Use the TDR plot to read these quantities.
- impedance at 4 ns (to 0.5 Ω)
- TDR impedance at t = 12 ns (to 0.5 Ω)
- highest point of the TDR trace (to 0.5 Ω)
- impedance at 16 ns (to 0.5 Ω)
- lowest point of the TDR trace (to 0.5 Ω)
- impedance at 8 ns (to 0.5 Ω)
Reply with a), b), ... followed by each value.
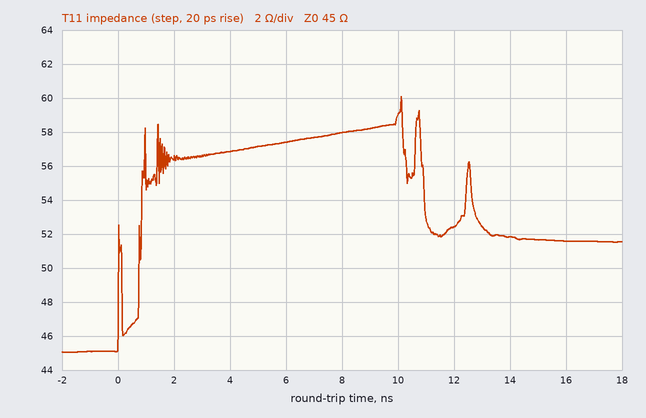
a) 57.0 Ω
b) 52.5 Ω
c) 60.0 Ω
d) 51.5 Ω
e) 45.0 Ω
f) 58.0 Ω
